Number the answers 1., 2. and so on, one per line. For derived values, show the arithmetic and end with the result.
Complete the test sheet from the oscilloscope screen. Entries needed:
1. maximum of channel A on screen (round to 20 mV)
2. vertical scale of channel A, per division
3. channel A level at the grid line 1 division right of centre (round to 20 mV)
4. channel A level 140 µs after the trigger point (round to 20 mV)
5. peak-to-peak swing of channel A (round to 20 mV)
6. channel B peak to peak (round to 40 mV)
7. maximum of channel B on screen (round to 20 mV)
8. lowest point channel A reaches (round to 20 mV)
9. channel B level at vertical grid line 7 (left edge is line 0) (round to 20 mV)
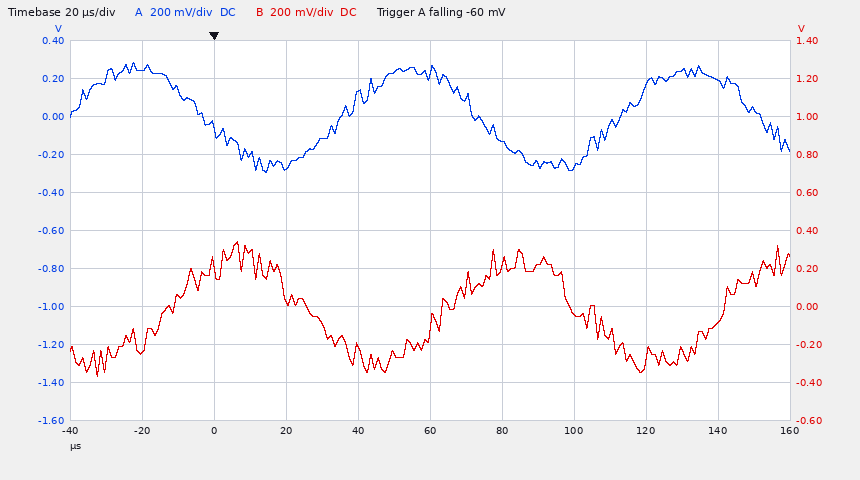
1. 280 mV
2. 200 mV
3. -140 mV
4. 180 mV
5. 280 mV − (-300 mV) = 580 mV
6. 720 mV
7. 340 mV
8. -300 mV
9. -40 mV
